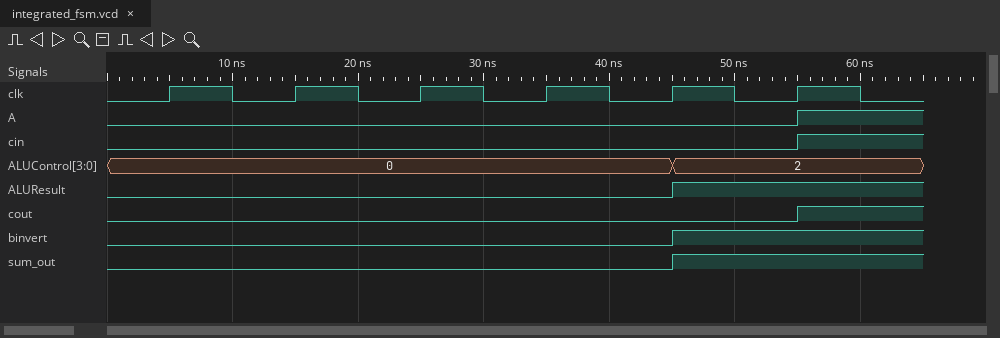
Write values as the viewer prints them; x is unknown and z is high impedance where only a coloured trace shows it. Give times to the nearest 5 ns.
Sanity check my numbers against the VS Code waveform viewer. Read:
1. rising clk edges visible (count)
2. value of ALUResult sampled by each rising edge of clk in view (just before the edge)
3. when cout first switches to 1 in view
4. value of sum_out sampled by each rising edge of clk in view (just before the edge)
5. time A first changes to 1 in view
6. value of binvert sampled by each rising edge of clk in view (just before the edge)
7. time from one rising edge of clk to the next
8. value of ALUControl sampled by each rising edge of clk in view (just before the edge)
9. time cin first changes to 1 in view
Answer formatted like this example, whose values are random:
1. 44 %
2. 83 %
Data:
1. 6
2. 0 0 0 0 0 1
3. 55 ns
4. 0 0 0 0 0 1
5. 55 ns
6. 0 0 0 0 0 1
7. 10 ns
8. 0, 0, 0, 0, 0, 2
9. 55 ns
